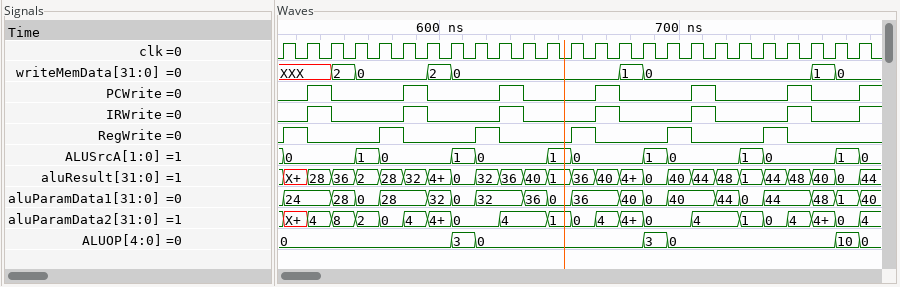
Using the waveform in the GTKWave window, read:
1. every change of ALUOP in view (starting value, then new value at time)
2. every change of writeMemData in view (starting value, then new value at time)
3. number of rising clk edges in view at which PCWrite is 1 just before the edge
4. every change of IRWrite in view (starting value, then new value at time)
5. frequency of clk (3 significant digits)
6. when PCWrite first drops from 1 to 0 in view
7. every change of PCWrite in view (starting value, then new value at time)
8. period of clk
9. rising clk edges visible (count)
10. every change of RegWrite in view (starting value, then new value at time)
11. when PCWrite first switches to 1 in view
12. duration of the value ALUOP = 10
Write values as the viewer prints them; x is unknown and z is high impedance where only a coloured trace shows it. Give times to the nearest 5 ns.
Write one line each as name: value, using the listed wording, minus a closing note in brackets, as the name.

every change of ALUOP in view: 0, 3 at 605 ns, 0 at 615 ns, 3 at 685 ns, 0 at 695 ns, 10 at 765 ns, 0 at 775 ns
every change of writeMemData in view: XXX, 2 at 555 ns, 0 at 565 ns, 2 at 595 ns, 0 at 605 ns, 1 at 675 ns, 0 at 685 ns, 1 at 755 ns, 0 at 765 ns
number of rising clk edges in view at which PCWrite is 1 just before the edge: 6
every change of IRWrite in view: 0, 1 at 545 ns, 0 at 555 ns, 1 at 585 ns, 0 at 595 ns, 1 at 625 ns, 0 at 635 ns, 1 at 665 ns, 0 at 675 ns, 1 at 705 ns, 0 at 715 ns, 1 at 745 ns, 0 at 755 ns, 1 at 775 ns
frequency of clk: 100 MHz
when PCWrite first drops from 1 to 0 in view: 555 ns
every change of PCWrite in view: 0, 1 at 545 ns, 0 at 555 ns, 1 at 585 ns, 0 at 595 ns, 1 at 625 ns, 0 at 635 ns, 1 at 665 ns, 0 at 675 ns, 1 at 705 ns, 0 at 715 ns, 1 at 745 ns, 0 at 755 ns, 1 at 775 ns
period of clk: 10 ns
rising clk edges visible: 25
every change of RegWrite in view: 0, 1 at 535 ns, 0 at 545 ns, 1 at 575 ns, 0 at 585 ns, 1 at 615 ns, 0 at 625 ns, 1 at 655 ns, 0 at 665 ns, 1 at 695 ns, 0 at 705 ns, 1 at 735 ns, 0 at 745 ns
when PCWrite first switches to 1 in view: 545 ns
duration of the value ALUOP = 10: 10 ns
